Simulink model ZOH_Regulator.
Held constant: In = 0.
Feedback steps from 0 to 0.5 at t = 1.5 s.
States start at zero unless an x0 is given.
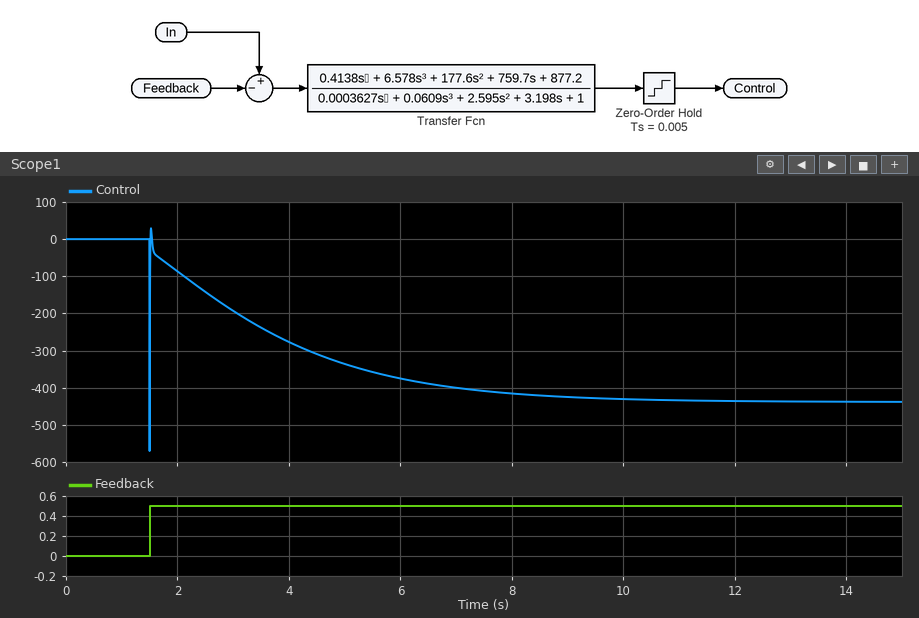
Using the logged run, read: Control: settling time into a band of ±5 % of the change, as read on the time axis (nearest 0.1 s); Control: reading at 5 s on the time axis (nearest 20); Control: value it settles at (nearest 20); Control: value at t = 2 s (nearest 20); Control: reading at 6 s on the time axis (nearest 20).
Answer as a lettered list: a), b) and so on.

a) 8.1 s
b) -340
c) -440
d) -80
e) -380
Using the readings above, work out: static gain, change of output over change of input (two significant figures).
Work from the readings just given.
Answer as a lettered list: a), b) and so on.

a) -880
